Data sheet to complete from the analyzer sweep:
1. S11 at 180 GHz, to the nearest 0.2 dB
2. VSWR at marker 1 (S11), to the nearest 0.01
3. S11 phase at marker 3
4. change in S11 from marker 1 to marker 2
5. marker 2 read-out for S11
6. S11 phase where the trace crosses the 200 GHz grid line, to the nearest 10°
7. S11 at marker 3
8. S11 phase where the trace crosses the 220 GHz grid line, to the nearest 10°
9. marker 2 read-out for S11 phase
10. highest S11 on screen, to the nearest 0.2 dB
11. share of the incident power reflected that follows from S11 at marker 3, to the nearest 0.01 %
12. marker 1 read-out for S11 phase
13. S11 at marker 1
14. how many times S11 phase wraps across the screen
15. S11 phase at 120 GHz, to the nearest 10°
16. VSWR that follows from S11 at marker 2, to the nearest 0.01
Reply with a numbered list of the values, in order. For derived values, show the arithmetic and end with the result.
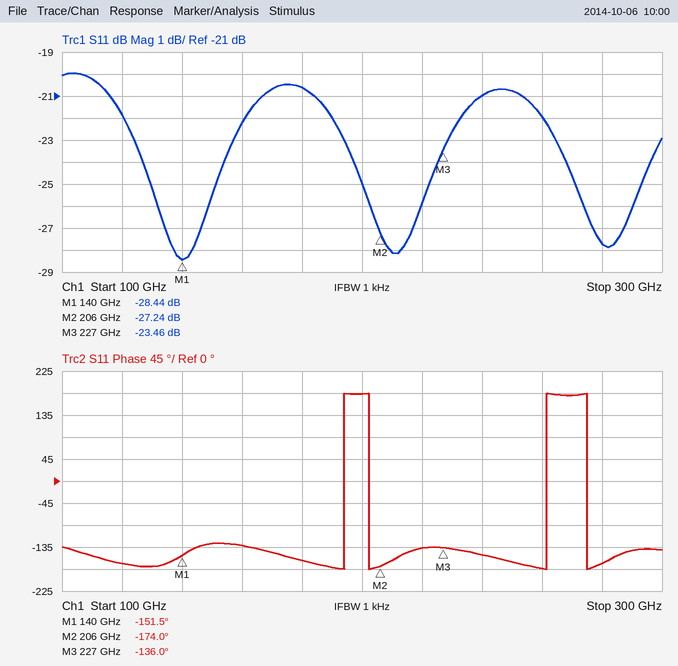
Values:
1. -20.6 dB
2. (1 + 0.0378)/(1 − 0.0378) ≈ 1.08
3. -136.0°
4. -27.24 − (-28.44) = 1.20 dB
5. -27.24 dB
6. 180°
7. -23.46 dB
8. -140°
9. -174.0°
10. -20.0 dB
11. 10^(-23.46/10) ≈ 0.45 %
12. -151.5°
13. -28.44 dB
14. 4
15. -170°
16. (1 + 0.0435)/(1 − 0.0435) ≈ 1.09
